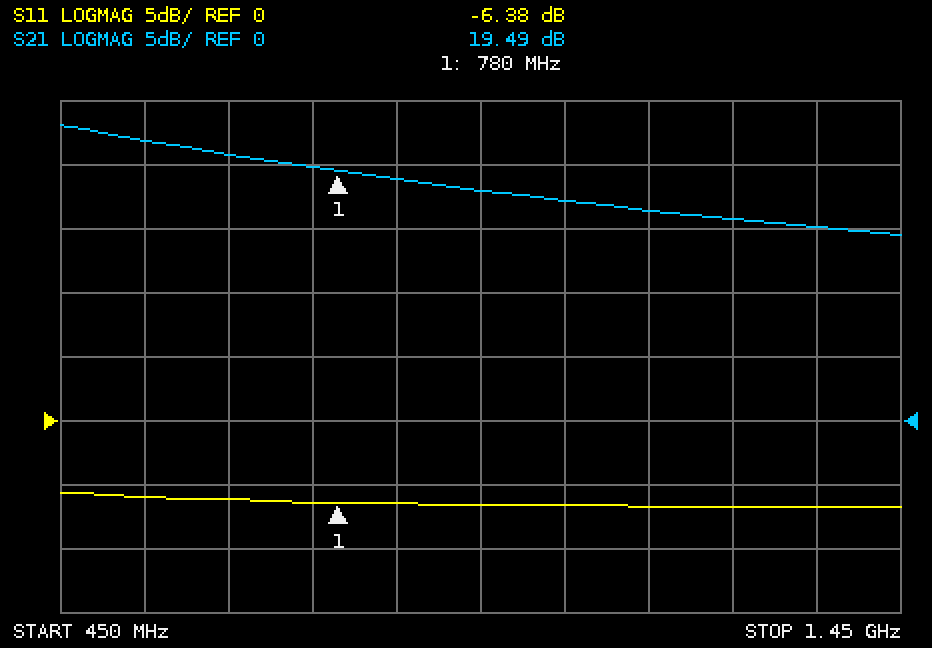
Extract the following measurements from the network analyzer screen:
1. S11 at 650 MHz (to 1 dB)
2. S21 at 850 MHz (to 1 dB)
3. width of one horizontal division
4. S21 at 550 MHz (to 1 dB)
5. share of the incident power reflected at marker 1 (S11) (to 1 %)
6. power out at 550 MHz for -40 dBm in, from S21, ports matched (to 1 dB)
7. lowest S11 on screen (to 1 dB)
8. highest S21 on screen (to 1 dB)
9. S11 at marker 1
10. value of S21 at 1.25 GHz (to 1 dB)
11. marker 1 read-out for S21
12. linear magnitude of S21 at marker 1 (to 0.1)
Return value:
-6 dB
19 dB
100 MHz
22 dB
23 %
-18 dBm
-7 dB
23 dB
-6.38 dB
16 dB
19.49 dB
9.4
